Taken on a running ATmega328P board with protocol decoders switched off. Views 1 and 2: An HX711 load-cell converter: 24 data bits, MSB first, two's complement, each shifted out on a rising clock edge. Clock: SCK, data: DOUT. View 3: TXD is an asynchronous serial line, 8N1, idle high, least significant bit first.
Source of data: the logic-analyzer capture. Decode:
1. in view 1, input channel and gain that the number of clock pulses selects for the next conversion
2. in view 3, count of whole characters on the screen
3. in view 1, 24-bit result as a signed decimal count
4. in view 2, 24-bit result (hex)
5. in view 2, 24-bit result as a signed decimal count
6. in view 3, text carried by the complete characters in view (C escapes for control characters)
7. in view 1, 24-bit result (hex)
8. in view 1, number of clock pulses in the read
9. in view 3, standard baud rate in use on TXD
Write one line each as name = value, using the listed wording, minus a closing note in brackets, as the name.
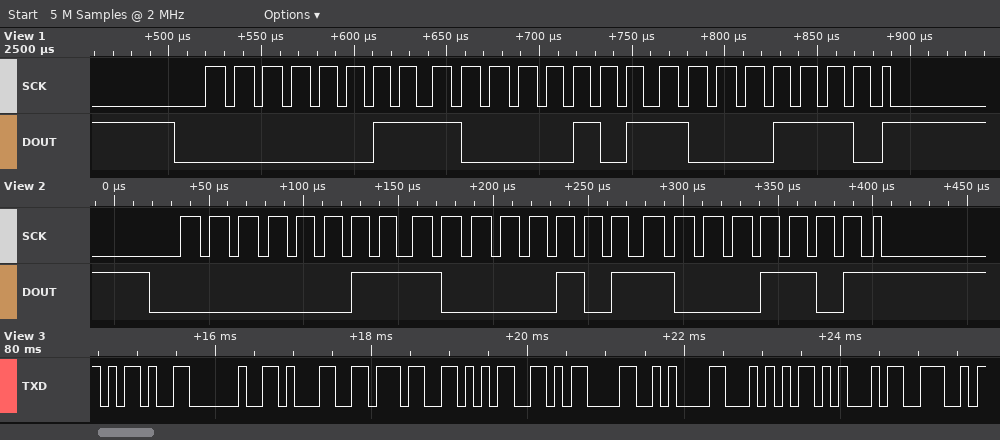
in view 1, input channel and gain that the number of clock pulses selects for the next conversion = channel A, gain 128
in view 3, count of whole characters on the screen = 10
in view 1, 24-bit result as a signed decimal count = 230798
in view 2, 24-bit result = 0x03858D
in view 2, 24-bit result as a signed decimal count = 230797
in view 3, text carried by the complete characters in view = "- 175\r\nTEN"
in view 1, 24-bit result = 0x03858E
in view 1, number of clock pulses in the read = 25
in view 3, standard baud rate in use on TXD = 9600 baud
